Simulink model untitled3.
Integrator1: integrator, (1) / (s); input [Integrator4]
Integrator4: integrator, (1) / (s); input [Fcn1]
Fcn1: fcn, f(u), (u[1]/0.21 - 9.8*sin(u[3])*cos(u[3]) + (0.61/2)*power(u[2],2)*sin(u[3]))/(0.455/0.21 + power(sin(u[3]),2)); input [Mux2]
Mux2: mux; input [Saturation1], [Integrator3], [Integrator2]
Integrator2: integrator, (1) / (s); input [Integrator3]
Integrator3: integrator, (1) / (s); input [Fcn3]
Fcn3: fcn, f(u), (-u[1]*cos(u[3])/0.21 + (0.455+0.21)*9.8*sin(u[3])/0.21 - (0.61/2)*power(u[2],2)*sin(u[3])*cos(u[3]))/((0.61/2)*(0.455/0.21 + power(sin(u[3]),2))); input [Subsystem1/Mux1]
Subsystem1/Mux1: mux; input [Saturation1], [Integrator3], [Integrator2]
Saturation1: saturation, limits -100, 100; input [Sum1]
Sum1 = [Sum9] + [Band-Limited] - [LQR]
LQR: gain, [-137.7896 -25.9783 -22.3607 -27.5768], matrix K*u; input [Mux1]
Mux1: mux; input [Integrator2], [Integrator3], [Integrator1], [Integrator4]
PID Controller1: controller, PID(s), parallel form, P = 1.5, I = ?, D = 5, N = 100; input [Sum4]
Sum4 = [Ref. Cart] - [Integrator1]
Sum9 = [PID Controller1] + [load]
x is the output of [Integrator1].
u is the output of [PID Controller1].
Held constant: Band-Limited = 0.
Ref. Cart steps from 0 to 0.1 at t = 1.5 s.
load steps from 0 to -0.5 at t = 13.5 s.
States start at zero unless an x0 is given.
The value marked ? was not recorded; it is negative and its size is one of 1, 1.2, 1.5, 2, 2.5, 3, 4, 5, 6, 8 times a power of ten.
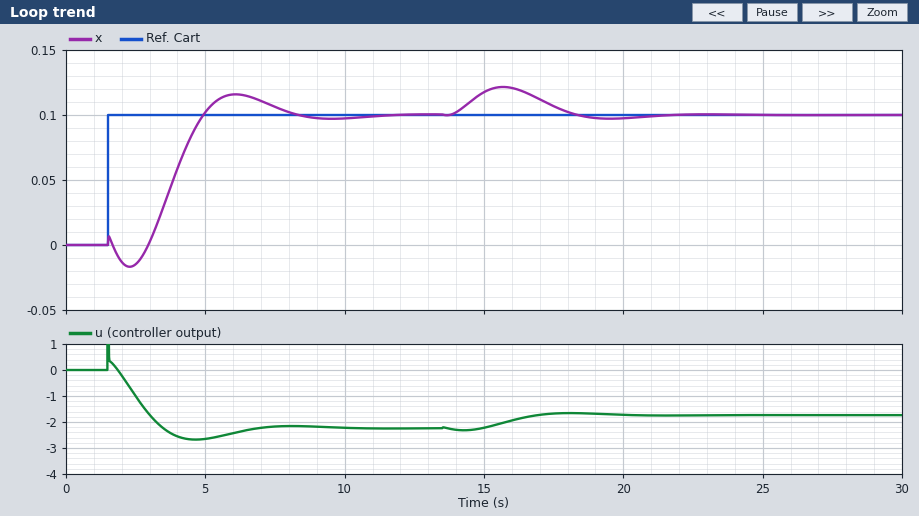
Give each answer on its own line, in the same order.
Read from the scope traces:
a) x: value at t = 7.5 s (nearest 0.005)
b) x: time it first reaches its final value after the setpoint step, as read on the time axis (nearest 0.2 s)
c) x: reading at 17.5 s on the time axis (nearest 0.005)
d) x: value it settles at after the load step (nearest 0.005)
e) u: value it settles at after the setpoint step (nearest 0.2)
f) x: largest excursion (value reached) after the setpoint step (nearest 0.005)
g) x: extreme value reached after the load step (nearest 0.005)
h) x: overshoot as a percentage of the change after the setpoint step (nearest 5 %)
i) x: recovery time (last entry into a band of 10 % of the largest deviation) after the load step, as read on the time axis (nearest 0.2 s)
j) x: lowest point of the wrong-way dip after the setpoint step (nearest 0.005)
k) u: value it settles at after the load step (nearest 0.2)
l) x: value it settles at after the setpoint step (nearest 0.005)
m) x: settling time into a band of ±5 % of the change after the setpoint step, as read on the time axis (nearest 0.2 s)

0.105
5.0 s
0.105
0.100
-2.2
0.115
0.120
15 %
20.4 s
-0.015
-1.8
0.100
7.6 s
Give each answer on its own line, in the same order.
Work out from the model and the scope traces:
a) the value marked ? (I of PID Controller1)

-10
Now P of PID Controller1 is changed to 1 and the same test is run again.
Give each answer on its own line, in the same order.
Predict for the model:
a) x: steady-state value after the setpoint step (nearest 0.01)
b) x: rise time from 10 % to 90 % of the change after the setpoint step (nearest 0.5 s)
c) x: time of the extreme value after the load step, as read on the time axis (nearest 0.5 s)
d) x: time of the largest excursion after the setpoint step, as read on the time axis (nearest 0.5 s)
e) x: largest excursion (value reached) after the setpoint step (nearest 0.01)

0.10
1.5 s
15.5 s
6.0 s
0.11
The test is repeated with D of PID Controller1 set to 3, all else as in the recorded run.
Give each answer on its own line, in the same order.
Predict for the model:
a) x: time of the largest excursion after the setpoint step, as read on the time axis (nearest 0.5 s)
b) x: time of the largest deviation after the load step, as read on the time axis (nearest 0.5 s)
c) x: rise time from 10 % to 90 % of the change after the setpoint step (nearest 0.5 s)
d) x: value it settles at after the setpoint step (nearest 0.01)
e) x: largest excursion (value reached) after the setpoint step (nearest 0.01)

6.5 s
15.5 s
2.0 s
0.10
0.11
